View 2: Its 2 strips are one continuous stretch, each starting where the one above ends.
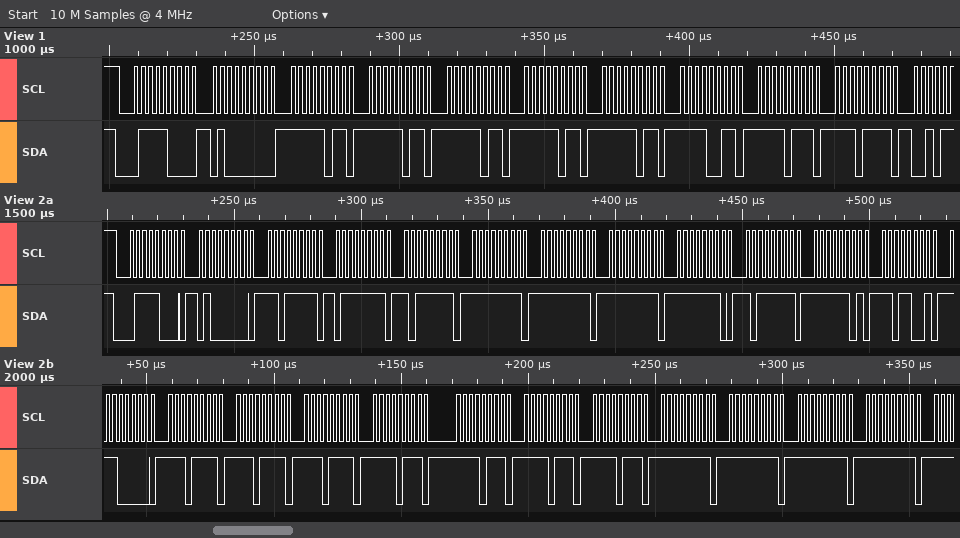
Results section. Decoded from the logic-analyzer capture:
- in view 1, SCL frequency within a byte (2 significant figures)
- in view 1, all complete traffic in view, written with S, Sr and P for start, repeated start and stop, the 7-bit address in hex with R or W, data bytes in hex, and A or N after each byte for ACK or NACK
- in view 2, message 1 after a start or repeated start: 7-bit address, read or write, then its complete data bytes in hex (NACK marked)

400 kHz
S 3CW A 40 A FB A FB A FB A FB A FB A F3 A F7 A EF A
0x3C write: 40 DF 7F BF FF FF FF FE BF FD D9 E0 EF EF EF F7 F7 F7 F7 FF FF FF FF
